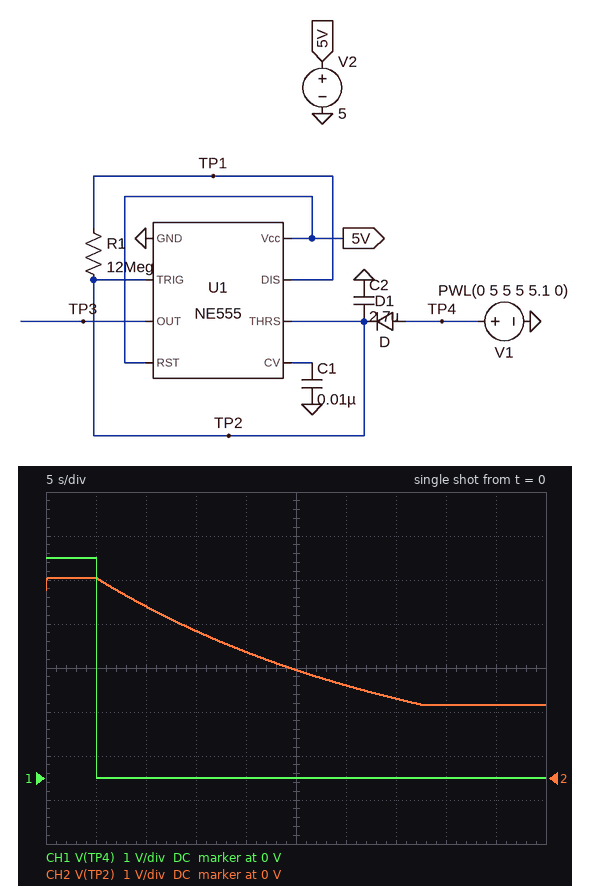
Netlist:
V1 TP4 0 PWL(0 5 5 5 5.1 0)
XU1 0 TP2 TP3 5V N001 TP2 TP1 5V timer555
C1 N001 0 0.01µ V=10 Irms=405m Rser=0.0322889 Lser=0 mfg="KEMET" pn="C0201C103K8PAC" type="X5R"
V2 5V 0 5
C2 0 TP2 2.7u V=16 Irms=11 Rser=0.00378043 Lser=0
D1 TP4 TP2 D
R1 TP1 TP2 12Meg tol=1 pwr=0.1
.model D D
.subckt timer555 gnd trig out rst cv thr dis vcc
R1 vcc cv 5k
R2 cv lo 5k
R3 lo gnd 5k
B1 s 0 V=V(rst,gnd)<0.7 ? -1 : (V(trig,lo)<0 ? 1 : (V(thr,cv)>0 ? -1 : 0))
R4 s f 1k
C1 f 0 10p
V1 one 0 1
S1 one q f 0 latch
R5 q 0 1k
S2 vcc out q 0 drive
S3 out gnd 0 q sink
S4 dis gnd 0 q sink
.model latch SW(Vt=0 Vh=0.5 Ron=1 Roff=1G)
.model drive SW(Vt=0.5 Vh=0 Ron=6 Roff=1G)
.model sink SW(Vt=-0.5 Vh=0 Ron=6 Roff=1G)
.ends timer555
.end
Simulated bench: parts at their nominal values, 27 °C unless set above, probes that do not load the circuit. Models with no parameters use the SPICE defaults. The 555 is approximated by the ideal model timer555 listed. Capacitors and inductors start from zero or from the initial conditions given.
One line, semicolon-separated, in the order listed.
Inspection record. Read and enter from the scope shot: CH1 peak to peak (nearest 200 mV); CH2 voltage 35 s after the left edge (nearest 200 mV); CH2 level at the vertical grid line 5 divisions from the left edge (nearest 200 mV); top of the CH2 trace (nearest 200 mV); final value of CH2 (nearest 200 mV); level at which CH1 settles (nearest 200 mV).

5.0 V; 1.8 V; 2.4 V; 4.6 V; 1.6 V; 0 V
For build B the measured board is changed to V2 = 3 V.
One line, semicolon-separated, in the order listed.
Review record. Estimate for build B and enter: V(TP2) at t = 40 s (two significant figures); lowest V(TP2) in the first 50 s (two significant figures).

1.5 V; 1.1 V
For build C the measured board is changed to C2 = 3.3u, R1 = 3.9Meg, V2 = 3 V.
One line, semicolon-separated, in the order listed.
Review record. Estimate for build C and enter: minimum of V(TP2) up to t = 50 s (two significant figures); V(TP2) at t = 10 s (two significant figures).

990 mV; 3.1 V
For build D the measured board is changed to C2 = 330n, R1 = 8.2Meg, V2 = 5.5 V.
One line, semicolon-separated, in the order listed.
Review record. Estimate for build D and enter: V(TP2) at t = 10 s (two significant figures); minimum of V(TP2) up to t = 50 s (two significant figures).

1.8 V; 1.6 V
